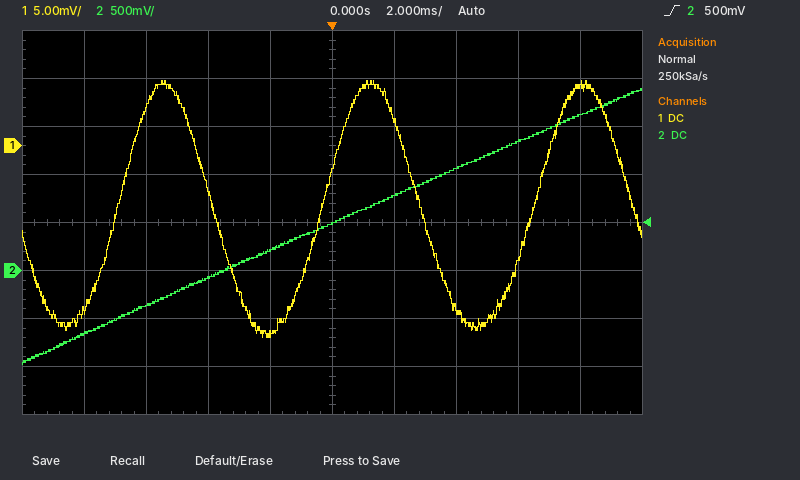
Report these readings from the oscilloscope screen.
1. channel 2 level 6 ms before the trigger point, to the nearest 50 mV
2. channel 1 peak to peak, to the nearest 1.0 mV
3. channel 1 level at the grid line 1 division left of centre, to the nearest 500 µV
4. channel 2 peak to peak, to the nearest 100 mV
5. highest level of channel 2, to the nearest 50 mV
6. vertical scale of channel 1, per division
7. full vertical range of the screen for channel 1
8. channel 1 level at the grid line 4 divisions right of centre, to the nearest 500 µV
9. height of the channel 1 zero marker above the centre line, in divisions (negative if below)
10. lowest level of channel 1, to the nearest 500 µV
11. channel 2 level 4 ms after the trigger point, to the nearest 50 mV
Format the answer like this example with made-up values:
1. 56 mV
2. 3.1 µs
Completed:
1. -350 mV
2. 27.0 mV
3. -19.5 mV
4. 2.90 V
5. 1.90 V
6. 5 mV
7. 40 mV
8. 6.5 mV
9. +1.6 div
10. -20.0 mV
11. 1.05 V
